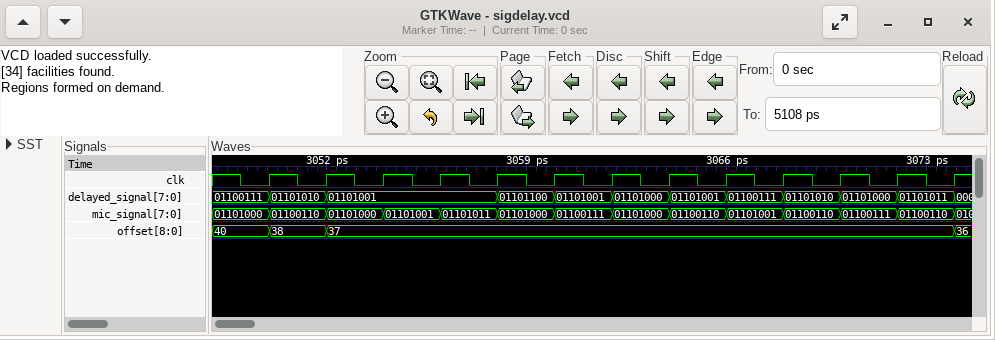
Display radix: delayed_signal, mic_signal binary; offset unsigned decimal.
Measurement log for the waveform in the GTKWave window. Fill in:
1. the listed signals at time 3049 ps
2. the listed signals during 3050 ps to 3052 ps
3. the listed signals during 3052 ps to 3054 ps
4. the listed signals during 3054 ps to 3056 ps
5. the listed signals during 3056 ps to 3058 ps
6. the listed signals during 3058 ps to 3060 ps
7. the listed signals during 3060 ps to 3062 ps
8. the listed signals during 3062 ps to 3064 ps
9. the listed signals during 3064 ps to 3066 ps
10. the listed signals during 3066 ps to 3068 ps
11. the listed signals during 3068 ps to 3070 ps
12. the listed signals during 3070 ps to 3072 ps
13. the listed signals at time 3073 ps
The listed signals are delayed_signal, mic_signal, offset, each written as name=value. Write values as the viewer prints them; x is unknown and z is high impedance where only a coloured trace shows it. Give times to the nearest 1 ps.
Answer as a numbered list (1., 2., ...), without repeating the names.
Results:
1. delayed_signal=01100111, mic_signal=01101000, offset=40
2. delayed_signal=01101010, mic_signal=01100110, offset=38
3. delayed_signal=01101001, mic_signal=01101000, offset=37
4. delayed_signal=01101001, mic_signal=01101001, offset=37
5. delayed_signal=01101001, mic_signal=01101011, offset=37
6. delayed_signal=01101100, mic_signal=01101000, offset=37
7. delayed_signal=01101001, mic_signal=01100111, offset=37
8. delayed_signal=01101000, mic_signal=01101000, offset=37
9. delayed_signal=01101001, mic_signal=01100110, offset=37
10. delayed_signal=01100111, mic_signal=01101001, offset=37
11. delayed_signal=01101010, mic_signal=01100110, offset=37
12. delayed_signal=01101000, mic_signal=01100111, offset=37
13. delayed_signal=01101011, mic_signal=01100110, offset=37
